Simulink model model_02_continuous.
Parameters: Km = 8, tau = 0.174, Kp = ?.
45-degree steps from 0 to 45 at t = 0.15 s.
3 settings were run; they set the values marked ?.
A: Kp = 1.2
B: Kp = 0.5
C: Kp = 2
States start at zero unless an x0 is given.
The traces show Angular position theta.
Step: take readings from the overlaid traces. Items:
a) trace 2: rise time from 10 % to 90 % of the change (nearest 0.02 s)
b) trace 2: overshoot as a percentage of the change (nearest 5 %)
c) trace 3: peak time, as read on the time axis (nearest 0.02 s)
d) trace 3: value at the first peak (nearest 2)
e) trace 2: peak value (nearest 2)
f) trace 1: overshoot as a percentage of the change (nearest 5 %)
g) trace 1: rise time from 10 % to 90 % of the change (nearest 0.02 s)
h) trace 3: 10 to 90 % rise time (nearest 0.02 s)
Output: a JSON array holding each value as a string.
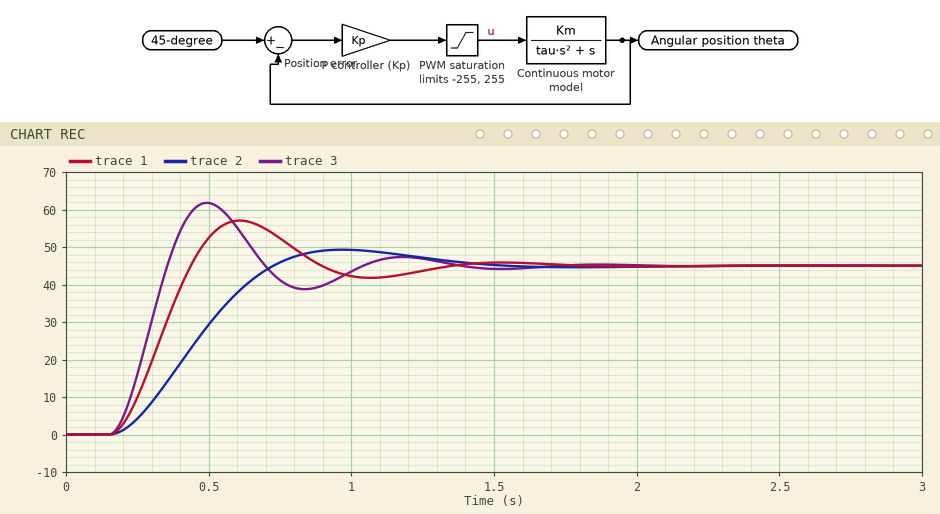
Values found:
["0.38 s", "10 %", "0.50 s", "62", "50", "25 %", "0.20 s", "0.14 s"]
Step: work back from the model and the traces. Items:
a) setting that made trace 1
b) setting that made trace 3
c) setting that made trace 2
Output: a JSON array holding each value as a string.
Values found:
["A", "C", "B"]
